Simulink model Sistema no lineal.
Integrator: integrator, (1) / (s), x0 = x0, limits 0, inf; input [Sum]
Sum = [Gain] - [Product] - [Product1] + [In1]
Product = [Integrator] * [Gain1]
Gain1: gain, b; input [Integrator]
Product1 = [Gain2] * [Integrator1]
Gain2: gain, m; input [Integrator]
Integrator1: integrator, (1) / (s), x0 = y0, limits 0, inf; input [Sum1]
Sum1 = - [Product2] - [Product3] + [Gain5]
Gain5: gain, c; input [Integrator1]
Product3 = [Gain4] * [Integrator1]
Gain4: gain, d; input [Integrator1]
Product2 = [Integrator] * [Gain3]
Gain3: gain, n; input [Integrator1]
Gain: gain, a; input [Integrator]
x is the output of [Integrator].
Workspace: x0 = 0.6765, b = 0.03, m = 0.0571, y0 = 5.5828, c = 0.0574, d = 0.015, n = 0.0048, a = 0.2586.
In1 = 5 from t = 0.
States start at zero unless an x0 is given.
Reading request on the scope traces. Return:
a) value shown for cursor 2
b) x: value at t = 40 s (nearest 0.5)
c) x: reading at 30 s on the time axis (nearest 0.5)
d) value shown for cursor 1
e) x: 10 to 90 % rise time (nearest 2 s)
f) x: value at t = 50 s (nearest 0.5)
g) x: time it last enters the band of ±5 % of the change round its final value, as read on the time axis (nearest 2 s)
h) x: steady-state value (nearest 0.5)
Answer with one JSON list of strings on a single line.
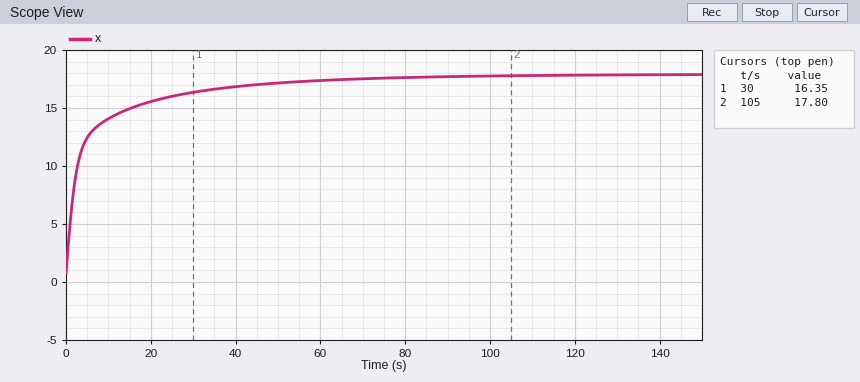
["17.80", "17.0", "16.5", "16.35", "28 s", "17.0", "46 s", "18.0"]
